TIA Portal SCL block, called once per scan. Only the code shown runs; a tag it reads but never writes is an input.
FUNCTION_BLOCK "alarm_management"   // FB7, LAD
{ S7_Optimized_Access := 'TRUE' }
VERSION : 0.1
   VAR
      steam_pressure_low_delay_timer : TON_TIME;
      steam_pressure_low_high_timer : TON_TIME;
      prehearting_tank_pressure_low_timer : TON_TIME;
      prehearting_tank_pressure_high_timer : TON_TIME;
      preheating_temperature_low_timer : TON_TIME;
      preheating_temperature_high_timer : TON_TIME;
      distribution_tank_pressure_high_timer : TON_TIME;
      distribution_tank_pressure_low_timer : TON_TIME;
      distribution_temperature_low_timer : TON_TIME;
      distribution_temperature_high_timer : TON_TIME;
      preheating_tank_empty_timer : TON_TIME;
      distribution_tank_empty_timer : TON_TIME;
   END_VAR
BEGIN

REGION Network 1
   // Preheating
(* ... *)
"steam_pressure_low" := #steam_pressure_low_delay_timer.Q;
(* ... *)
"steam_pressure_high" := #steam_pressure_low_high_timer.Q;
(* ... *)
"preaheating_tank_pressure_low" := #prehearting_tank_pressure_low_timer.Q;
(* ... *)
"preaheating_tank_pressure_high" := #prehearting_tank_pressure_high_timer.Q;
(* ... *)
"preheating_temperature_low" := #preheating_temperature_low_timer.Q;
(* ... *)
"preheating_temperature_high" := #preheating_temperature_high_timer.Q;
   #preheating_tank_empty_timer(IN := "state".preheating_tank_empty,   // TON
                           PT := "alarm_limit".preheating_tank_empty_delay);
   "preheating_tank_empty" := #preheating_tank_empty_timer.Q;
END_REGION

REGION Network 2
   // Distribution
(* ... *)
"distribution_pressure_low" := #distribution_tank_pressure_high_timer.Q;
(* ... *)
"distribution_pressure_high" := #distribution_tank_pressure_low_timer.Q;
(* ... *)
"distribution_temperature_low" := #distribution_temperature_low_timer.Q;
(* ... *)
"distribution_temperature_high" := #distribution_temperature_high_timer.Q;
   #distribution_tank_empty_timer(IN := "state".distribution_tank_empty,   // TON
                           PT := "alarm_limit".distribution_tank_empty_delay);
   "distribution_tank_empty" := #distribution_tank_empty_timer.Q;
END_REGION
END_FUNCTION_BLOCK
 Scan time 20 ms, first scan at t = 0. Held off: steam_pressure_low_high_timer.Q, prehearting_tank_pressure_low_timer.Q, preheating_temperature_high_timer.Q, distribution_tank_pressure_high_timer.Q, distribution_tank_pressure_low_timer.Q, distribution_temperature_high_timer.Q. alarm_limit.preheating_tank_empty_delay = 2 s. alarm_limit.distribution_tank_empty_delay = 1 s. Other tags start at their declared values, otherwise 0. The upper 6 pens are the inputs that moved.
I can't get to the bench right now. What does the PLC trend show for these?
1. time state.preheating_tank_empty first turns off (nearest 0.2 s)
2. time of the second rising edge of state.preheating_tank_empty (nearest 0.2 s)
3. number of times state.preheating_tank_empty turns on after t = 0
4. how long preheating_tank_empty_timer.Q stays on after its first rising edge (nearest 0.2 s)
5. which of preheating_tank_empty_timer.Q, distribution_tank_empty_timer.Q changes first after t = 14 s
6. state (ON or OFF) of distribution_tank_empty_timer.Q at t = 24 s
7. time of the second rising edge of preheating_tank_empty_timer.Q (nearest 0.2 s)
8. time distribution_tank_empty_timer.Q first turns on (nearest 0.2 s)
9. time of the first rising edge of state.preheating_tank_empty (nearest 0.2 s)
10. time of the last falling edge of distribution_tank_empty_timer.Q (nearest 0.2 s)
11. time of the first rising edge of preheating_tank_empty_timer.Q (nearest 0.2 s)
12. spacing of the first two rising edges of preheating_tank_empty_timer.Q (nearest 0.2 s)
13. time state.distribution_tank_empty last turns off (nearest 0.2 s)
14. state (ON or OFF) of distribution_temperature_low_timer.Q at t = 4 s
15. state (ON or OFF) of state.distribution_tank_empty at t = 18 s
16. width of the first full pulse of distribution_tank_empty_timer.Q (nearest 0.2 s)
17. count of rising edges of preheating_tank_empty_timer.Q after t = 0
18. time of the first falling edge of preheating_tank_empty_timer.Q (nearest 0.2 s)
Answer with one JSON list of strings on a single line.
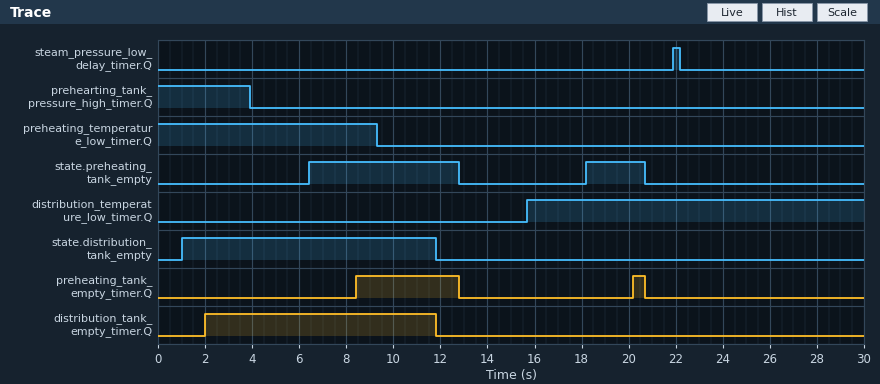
["12.8 s", "18.2 s", "2", "4.4 s", "preheating_tank_empty_timer.Q", "OFF", "20.2 s", "2.0 s", "6.4 s", "11.8 s", "8.4 s", "11.8 s", "11.8 s", "OFF", "OFF", "9.8 s", "2", "12.8 s"]
